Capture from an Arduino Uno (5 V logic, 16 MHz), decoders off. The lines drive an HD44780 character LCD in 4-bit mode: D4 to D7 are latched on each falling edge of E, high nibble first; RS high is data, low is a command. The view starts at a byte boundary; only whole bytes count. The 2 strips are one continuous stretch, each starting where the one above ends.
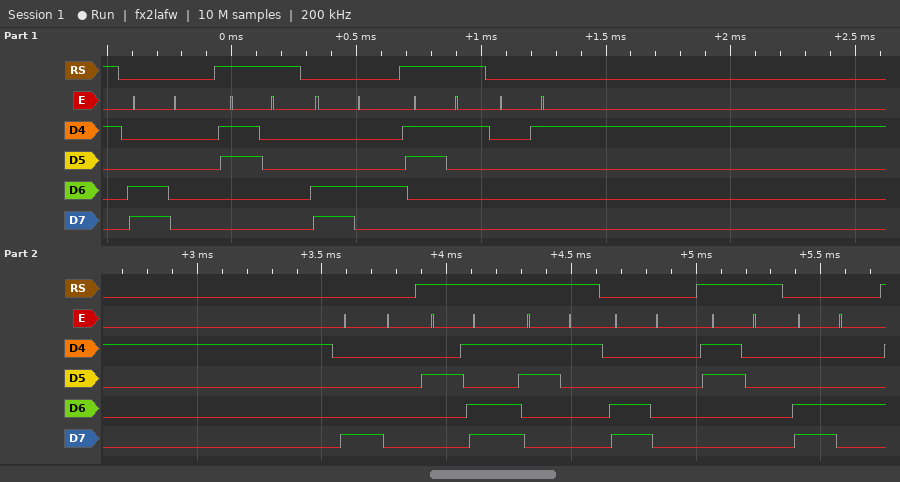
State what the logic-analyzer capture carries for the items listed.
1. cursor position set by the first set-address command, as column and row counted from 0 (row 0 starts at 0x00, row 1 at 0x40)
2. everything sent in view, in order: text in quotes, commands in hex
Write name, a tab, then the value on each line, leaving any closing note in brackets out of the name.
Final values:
cursor position set by the first set-address command, as column and row counted from 0	column 0, row 1
everything sent in view, in order: text in quotes, commands in hex	0xC0 "0" 0xC4 "1" 0x01 0x80 "-1" 0xC0 "0" 0xC4
